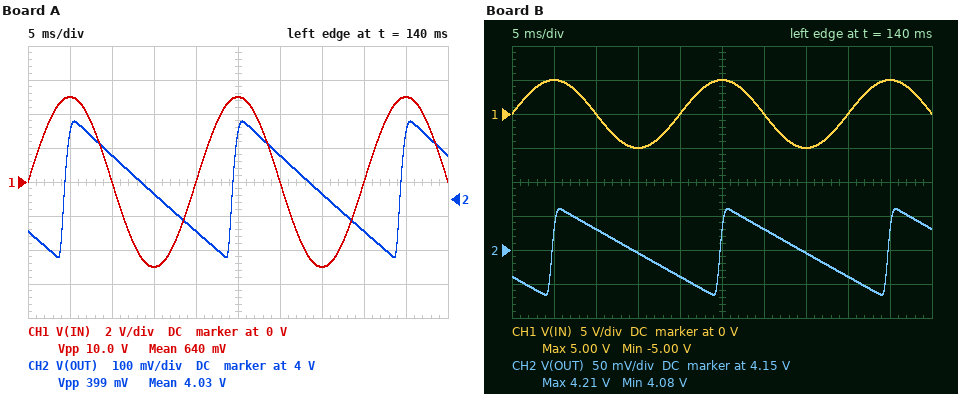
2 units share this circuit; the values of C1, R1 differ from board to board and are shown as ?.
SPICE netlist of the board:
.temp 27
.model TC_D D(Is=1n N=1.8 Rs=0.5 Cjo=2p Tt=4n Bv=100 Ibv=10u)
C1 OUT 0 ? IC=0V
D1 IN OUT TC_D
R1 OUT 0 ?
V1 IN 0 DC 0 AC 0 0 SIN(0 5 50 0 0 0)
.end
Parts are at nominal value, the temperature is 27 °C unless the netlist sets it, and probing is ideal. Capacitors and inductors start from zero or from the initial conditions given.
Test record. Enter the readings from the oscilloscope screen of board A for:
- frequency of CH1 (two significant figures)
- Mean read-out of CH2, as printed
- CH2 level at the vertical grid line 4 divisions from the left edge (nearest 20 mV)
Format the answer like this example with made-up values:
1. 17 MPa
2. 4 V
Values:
1. 50 Hz
2. 4.03 V
3. 3.90 V
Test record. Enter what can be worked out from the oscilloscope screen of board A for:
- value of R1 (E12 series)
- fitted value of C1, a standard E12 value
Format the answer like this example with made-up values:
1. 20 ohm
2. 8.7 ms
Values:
1. 1.2 kΩ
2. 150 µF
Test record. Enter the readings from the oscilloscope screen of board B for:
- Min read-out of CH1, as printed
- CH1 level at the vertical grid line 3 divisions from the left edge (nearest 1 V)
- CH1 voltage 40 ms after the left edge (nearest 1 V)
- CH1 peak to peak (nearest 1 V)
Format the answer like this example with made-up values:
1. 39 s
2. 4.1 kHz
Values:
1. -5.00 V
2. -5 V
3. 0 V
4. 10 V
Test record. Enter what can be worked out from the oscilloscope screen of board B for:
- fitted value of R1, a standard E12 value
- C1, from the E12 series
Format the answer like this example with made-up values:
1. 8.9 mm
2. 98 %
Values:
1. 2.2 kΩ
2. 270 µF
